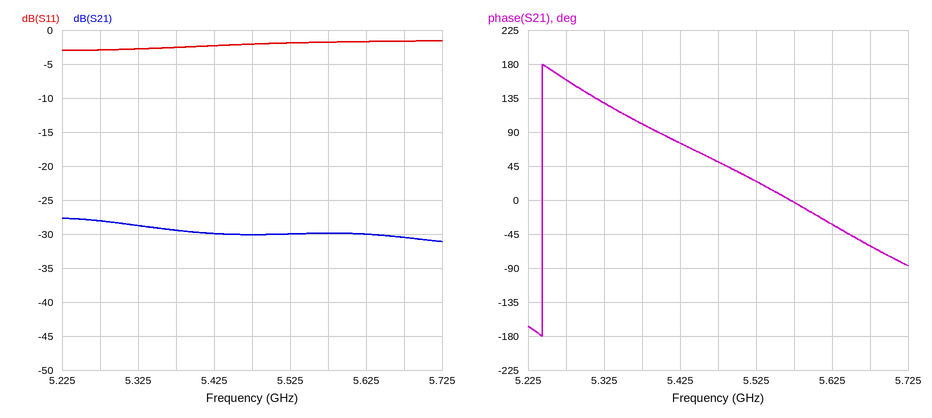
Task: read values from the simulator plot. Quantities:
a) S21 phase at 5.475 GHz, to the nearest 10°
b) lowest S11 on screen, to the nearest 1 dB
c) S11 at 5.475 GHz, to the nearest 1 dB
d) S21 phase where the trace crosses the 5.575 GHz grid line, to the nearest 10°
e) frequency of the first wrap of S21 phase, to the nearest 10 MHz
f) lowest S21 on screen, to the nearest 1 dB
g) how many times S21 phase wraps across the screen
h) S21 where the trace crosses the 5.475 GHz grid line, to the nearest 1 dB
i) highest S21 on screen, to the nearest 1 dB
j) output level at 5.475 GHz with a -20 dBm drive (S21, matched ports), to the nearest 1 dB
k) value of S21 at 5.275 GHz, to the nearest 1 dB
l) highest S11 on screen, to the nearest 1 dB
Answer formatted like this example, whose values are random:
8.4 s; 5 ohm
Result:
50°; -3 dB; -2 dB; 0°; 5.24 GHz; -31 dB; 1; -30 dB; -28 dB; -50 dBm; -28 dB; -2 dB
